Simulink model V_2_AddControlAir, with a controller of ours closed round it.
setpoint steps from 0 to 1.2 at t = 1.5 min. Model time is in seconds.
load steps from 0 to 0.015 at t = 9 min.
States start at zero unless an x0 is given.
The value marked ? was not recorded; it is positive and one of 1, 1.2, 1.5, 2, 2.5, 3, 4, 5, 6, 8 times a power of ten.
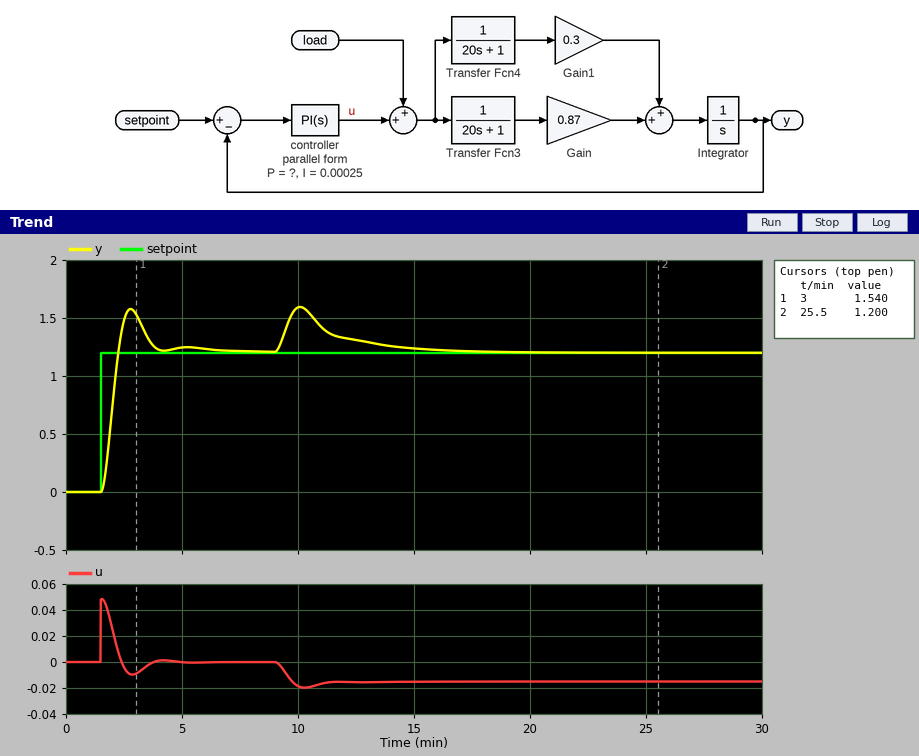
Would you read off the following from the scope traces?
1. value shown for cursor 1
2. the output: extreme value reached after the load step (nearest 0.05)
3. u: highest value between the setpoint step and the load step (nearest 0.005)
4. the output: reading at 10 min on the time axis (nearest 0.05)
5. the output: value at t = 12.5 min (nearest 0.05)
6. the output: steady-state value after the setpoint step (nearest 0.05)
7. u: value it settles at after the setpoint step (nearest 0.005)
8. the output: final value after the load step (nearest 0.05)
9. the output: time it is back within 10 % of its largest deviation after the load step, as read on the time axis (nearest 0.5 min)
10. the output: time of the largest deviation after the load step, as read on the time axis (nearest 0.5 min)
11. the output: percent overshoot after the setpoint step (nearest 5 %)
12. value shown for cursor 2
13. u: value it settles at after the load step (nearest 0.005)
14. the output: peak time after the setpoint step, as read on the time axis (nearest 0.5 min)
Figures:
1.540
1.60
0.050
1.60
1.30
1.20
0.000
1.20
15.0 min
10.0 min
30 %
1.200
-0.015
3.0 min
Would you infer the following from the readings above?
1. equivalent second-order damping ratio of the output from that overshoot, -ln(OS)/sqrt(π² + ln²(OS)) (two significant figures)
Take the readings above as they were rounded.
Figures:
0.36
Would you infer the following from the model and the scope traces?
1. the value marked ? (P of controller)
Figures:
0.04
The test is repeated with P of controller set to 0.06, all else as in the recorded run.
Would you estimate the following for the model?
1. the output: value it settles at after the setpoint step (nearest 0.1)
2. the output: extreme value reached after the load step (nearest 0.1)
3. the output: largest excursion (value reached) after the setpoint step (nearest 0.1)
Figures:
1.2
1.5
1.6
